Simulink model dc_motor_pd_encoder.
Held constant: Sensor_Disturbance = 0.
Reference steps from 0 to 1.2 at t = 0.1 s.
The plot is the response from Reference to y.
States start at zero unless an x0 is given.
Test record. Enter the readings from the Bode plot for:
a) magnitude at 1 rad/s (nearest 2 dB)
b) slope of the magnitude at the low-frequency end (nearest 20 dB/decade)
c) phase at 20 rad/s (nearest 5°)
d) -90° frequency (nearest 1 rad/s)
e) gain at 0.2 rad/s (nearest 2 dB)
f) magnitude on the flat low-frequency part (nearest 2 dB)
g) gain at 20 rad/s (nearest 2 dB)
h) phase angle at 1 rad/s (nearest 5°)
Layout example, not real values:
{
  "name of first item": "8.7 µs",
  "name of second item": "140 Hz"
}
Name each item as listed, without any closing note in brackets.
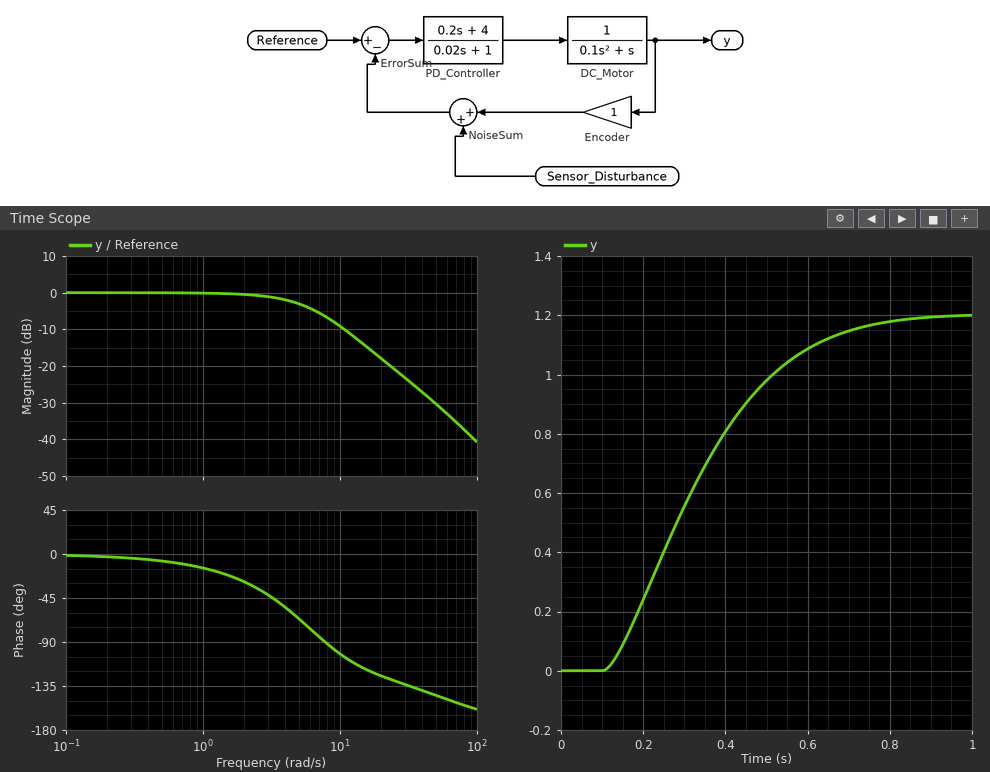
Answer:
{
  "magnitude at 1 rad/s": "0 dB",
  "slope of the magnitude at the low-frequency end": "0 dB/decade",
  "phase at 20 rad/s": "-125°",
  "-90° frequency": "8 rad/s",
  "gain at 0.2 rad/s": "0 dB",
  "magnitude on the flat low-frequency part": "0 dB",
  "gain at 20 rad/s": "-18 dB",
  "phase angle at 1 rad/s": "-15°"
}
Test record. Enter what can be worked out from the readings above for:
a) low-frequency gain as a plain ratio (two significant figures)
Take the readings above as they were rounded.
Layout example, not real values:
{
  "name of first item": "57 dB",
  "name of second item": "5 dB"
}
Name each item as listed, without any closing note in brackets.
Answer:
{
  "low-frequency gain as a plain ratio": "1.0"
}
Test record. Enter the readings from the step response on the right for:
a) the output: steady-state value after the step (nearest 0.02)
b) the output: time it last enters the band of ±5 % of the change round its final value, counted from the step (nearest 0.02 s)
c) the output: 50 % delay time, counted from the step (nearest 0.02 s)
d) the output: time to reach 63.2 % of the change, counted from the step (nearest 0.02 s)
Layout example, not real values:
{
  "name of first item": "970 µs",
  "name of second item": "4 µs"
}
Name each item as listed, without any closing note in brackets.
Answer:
{
  "the output: steady-state value after the step": "1.20",
  "the output: time it last enters the band of ±5 % of the change round its final value, counted from the step": "0.58 s",
  "the output: 50 % delay time, counted from the step": "0.22 s",
  "the output: time to reach 63.2 % of the change, counted from the step": "0.28 s"
}
